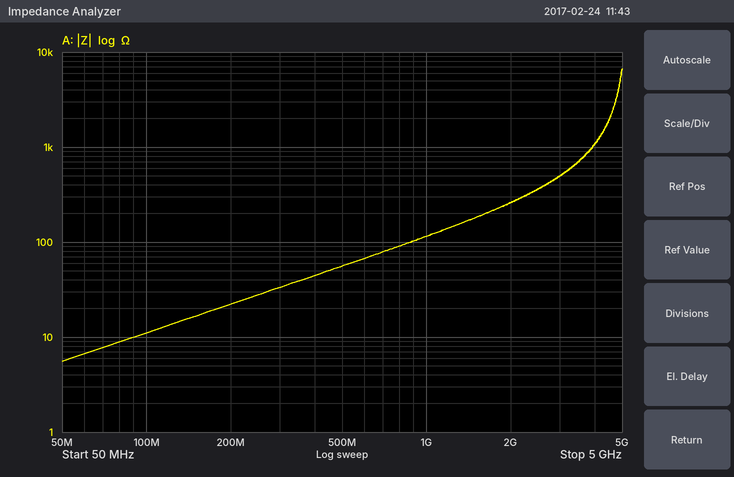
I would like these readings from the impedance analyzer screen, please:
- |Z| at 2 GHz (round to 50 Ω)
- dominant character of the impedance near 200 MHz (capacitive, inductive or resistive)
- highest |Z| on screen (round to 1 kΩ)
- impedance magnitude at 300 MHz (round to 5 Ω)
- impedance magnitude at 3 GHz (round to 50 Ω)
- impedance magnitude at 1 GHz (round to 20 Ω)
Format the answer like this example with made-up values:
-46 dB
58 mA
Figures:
250 Ω
inductive
7 kΩ
35 Ω
500 Ω
120 Ω
